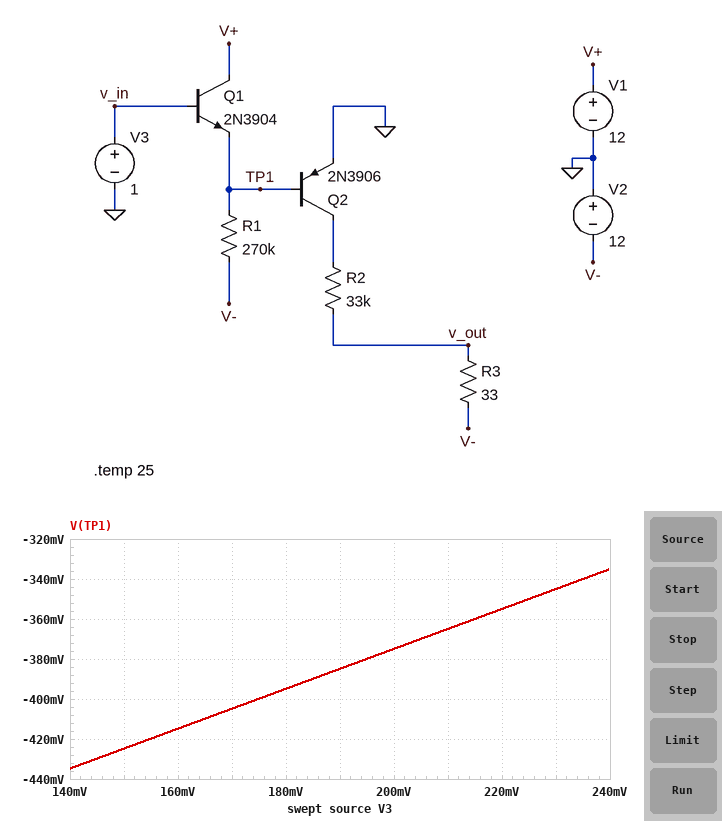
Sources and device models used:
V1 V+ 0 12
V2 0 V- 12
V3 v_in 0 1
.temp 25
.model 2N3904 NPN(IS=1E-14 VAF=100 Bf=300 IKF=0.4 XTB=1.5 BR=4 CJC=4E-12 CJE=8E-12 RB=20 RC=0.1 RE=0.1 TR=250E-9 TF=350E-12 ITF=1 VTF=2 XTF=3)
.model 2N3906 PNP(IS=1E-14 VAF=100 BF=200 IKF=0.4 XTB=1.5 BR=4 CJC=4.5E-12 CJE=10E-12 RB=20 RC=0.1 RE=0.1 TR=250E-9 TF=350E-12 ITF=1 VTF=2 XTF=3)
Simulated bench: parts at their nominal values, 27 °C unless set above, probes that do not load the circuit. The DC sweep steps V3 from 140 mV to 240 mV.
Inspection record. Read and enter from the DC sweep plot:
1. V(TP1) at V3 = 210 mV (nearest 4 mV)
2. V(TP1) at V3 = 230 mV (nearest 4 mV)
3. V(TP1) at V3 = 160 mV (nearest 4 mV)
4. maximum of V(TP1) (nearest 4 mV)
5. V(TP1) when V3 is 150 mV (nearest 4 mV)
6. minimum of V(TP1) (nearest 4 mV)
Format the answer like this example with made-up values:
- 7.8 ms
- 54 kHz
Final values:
- -364 mV
- -344 mV
- -416 mV
- -336 mV
- -424 mV
- -436 mV
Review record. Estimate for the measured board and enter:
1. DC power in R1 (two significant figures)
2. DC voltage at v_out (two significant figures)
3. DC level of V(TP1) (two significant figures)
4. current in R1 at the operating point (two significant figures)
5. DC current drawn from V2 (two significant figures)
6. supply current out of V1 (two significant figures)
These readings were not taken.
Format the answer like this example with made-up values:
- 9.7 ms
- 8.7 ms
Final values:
- 570 µW
- -12 V
- 420 mV
- 46 µA
- 46 µA
- 46 µA
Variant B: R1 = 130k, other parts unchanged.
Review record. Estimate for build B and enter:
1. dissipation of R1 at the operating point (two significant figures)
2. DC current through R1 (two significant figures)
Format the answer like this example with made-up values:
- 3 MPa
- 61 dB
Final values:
- 1.2 mW
- 95 µA
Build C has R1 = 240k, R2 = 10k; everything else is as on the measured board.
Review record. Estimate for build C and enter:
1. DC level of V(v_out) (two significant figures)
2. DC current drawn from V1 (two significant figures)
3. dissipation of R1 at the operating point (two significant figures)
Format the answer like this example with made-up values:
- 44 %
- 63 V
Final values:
- -12 V
- 52 µA
- 640 µW
